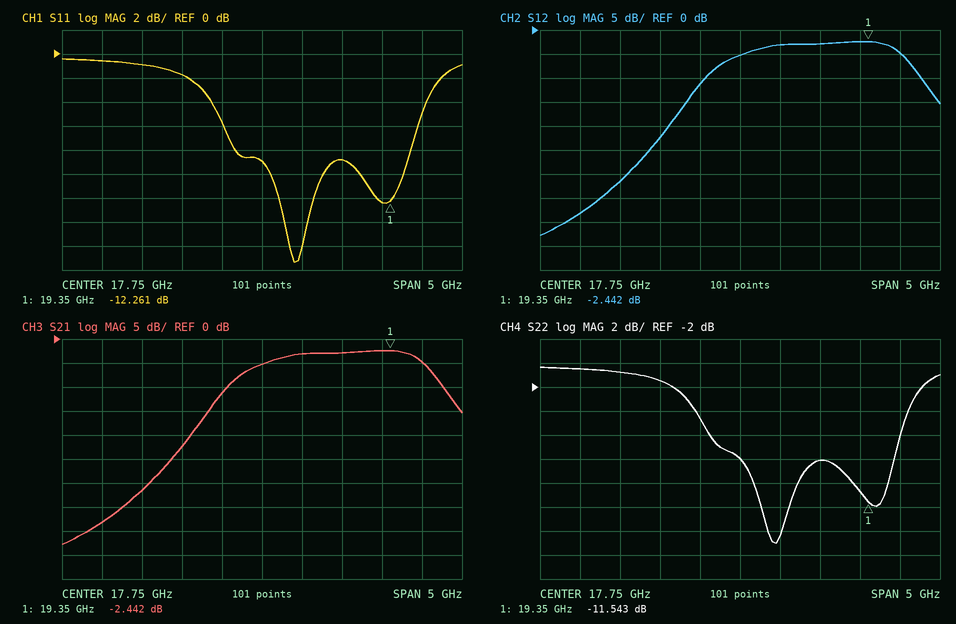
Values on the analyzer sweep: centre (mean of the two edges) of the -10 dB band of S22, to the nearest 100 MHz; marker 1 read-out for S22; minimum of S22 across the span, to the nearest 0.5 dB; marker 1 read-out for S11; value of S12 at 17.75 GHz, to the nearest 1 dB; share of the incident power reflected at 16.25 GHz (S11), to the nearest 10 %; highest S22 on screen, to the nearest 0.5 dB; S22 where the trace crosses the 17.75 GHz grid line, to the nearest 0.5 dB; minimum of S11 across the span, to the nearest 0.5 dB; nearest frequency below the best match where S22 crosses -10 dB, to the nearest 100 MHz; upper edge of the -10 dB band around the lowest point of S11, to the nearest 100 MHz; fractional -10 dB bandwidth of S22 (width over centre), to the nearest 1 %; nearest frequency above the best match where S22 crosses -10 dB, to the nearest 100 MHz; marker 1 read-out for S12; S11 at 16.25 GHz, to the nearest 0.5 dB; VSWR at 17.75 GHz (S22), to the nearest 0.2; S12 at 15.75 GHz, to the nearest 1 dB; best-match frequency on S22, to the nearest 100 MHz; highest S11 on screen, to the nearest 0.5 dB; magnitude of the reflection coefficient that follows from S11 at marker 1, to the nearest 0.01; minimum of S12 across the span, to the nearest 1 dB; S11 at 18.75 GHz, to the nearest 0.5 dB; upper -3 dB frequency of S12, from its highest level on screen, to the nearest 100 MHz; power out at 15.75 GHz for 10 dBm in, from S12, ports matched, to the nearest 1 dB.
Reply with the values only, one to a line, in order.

18.2 GHz
-11.543 dB
-15.0 dB
-12.261 dB
-5 dB
80 %
-0.5 dB
-8.0 dB
-17.5 dB
17.9 GHz
18.5 GHz
3 %
18.5 GHz
-2.442 dB
-1.0 dB
2.4
-38 dB
18.2 GHz
-0.5 dB
0.24
-43 dB
-9.0 dB
19.8 GHz
-28 dBm
